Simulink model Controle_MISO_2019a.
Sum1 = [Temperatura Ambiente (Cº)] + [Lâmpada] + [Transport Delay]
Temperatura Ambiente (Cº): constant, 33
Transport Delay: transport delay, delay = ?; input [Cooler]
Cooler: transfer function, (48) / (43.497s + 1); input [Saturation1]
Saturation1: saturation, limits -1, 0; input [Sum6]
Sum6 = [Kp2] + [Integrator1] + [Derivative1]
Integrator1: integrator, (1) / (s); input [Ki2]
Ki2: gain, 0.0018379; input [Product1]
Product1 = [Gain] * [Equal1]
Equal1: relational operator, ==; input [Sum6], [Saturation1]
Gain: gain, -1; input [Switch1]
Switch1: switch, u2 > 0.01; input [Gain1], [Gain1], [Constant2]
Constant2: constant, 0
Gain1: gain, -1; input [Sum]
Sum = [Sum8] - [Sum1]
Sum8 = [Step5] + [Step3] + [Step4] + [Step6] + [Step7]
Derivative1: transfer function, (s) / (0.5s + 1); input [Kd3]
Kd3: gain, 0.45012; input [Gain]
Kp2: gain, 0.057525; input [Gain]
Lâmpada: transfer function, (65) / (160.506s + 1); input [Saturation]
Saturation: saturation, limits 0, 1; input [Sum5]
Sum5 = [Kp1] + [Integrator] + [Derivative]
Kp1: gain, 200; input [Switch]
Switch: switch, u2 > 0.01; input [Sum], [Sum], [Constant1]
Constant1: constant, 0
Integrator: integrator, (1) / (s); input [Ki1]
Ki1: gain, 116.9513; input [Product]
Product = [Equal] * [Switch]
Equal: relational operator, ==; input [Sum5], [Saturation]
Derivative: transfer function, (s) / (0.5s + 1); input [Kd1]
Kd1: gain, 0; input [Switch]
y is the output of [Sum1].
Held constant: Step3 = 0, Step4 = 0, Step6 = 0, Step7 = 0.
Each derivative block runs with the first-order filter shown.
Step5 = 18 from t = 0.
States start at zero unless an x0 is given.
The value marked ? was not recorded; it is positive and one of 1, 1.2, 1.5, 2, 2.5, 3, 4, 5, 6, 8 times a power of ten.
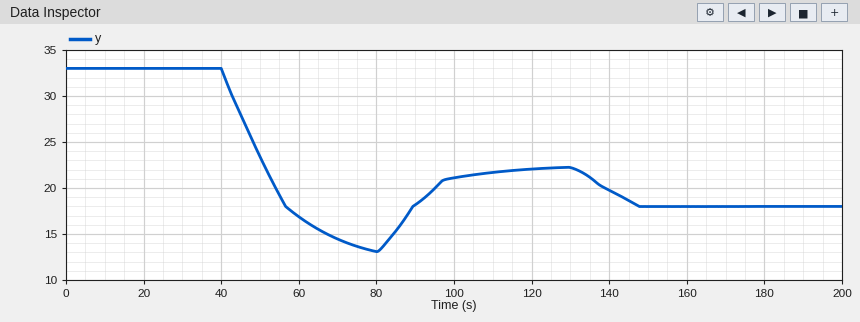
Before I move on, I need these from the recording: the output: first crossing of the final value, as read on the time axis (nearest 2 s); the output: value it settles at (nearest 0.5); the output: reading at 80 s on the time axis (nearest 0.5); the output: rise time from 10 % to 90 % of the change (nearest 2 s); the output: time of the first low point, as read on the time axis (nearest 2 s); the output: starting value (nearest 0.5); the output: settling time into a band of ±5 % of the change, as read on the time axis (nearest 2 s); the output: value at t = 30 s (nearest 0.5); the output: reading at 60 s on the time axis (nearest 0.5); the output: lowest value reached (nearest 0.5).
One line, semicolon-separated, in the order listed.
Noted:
56 s; 18.0; 13.0; 14 s; 80 s; 33.0; 144 s; 33.0; 17.0; 13.0
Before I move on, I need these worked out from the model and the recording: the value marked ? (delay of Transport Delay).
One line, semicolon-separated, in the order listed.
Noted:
40
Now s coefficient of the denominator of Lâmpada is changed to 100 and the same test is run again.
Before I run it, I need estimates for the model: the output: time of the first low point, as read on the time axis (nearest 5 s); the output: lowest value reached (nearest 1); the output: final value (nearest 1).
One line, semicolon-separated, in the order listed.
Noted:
70 s; 17; 18
